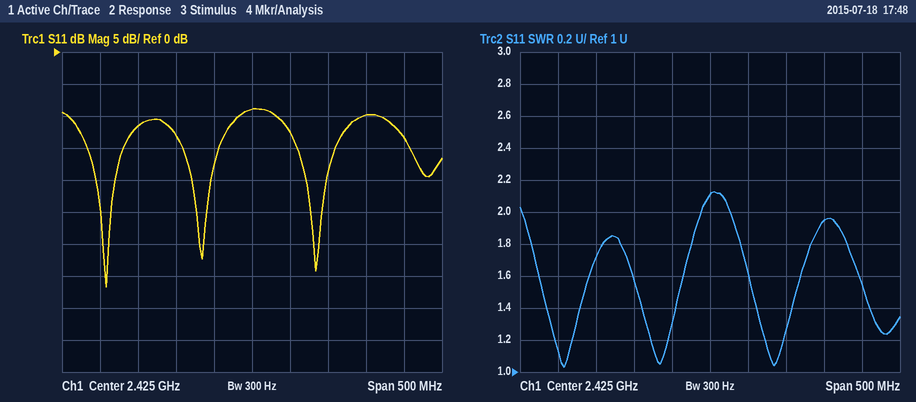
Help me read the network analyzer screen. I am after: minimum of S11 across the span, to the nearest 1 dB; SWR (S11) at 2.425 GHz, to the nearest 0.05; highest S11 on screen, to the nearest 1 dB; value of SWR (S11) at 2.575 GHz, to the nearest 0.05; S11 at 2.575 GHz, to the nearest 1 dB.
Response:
-37 dB
2.10
-9 dB
1.95
-10 dB
